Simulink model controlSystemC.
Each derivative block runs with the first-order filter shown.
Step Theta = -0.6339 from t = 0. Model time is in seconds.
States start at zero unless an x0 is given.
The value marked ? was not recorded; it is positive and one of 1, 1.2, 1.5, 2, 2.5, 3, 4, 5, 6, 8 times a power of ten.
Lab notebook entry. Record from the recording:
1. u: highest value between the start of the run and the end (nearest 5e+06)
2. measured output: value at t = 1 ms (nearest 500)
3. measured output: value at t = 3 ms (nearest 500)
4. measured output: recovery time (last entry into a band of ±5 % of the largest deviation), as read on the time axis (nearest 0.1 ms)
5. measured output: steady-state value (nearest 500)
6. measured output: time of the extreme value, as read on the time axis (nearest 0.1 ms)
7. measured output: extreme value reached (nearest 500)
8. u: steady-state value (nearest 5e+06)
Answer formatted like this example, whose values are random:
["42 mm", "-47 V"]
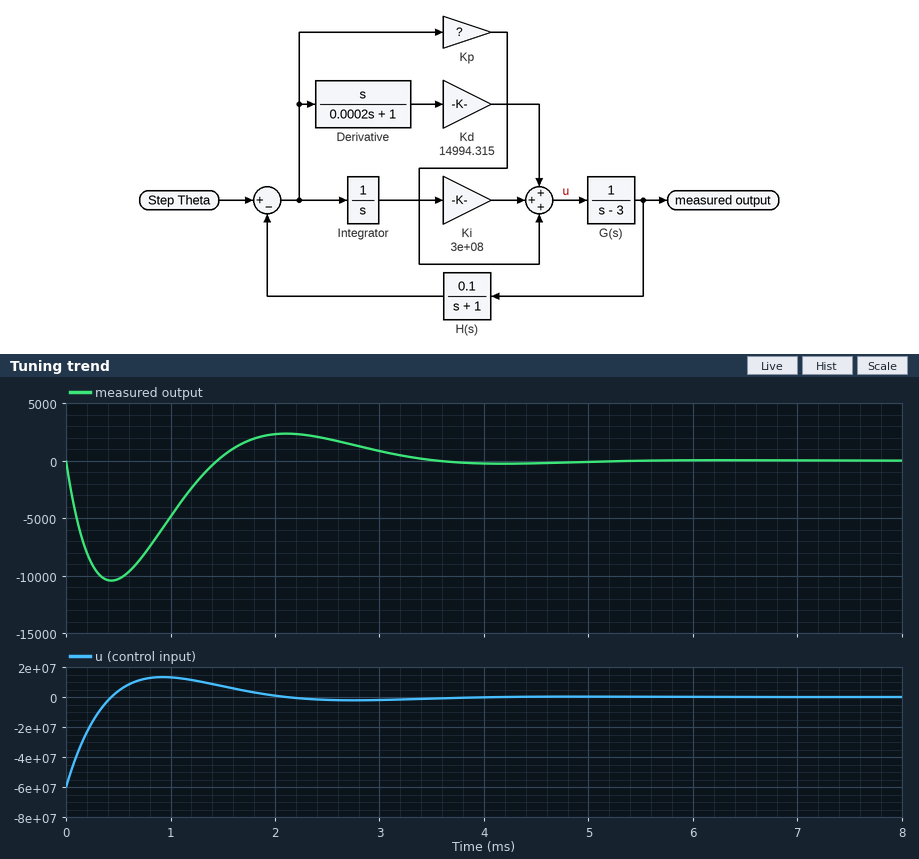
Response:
["15000000", "-5000", "1000", "3.2 ms", "0", "0.4 ms", "-10500", "0"]
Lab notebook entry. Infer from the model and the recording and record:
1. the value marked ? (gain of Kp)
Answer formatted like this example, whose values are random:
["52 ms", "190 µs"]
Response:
["2e+07"]
